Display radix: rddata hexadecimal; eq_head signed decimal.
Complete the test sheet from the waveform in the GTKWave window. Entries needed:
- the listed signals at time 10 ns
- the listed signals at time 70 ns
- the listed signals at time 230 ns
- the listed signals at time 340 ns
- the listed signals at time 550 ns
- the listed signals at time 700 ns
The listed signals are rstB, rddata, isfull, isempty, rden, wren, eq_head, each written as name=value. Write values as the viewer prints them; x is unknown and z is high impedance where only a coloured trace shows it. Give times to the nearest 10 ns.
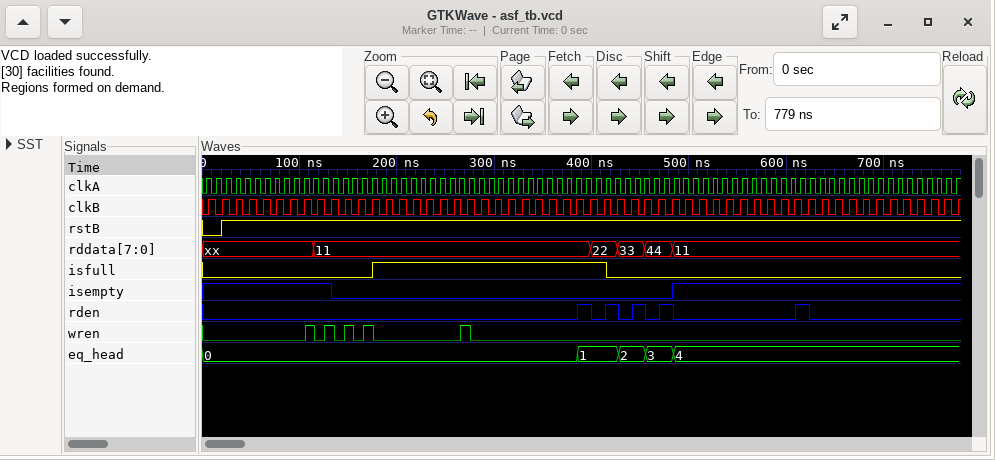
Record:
rstB=0, rddata=xx, isfull=0, isempty=1, rden=0, wren=0, eq_head=0
rstB=1, rddata=xx, isfull=0, isempty=1, rden=0, wren=0, eq_head=0
rstB=1, rddata=11, isfull=1, isempty=0, rden=0, wren=0, eq_head=0
rstB=1, rddata=11, isfull=1, isempty=0, rden=0, wren=0, eq_head=0
rstB=1, rddata=11, isfull=0, isempty=1, rden=0, wren=0, eq_head=4
rstB=1, rddata=11, isfull=0, isempty=1, rden=0, wren=0, eq_head=4
